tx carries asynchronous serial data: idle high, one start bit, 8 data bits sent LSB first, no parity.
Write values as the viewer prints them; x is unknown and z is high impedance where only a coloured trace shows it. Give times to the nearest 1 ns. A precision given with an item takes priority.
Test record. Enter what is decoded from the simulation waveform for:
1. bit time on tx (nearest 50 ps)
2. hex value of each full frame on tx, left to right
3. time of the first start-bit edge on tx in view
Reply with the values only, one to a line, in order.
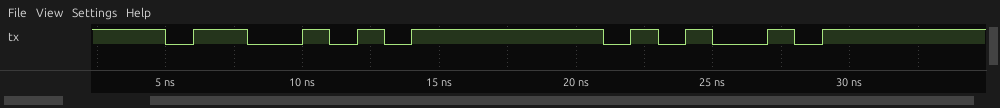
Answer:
1000 ps
53, A5
5 ns
